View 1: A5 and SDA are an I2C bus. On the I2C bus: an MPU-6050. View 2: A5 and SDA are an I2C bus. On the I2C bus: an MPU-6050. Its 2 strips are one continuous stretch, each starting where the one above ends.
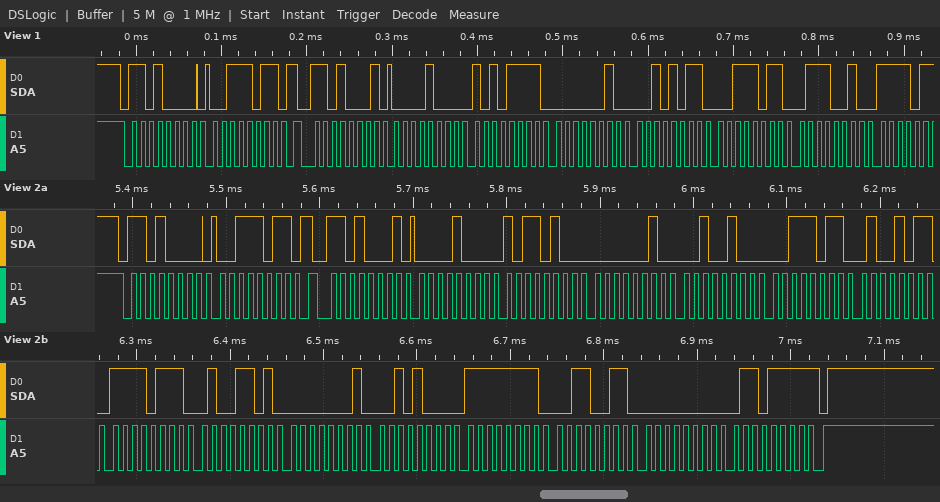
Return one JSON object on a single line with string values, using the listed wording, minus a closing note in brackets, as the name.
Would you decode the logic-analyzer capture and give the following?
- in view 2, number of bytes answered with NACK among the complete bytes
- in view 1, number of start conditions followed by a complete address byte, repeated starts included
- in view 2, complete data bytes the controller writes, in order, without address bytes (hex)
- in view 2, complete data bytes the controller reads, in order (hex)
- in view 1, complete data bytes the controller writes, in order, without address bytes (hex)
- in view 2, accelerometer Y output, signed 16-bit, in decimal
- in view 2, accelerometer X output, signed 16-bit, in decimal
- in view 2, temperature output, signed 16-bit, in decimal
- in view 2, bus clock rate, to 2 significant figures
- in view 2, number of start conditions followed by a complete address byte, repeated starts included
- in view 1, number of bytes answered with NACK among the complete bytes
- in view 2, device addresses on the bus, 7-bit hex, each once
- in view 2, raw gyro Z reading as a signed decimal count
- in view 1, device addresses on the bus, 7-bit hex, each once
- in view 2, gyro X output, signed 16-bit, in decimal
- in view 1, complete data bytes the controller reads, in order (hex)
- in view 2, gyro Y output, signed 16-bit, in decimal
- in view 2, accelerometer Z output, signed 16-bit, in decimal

{"in view 2, number of bytes answered with NACK among the complete bytes": "1", "in view 1, number of start conditions followed by a complete address byte, repeated starts included": "2", "in view 2, complete data bytes the controller writes, in order, without address bytes": "3B", "in view 2, complete data bytes the controller reads, in order": "08 B4 02 24 3B 4B F7 4D 01 28 FF 33 00 6F", "in view 1, complete data bytes the controller writes, in order, without address bytes": "3B", "in view 2, accelerometer Y output, signed 16-bit, in decimal": "548", "in view 2, accelerometer X output, signed 16-bit, in decimal": "2228", "in view 2, temperature output, signed 16-bit, in decimal": "-2227", "in view 2, bus clock rate, to 2 significant figures": "100 kHz", "in view 2, number of start conditions followed by a complete address byte, repeated starts included": "2", "in view 1, number of bytes answered with NACK among the complete bytes": "0", "in view 2, device addresses on the bus, 7-bit hex, each once": "0x68", "in view 2, raw gyro Z reading as a signed decimal count": "111", "in view 1, device addresses on the bus, 7-bit hex, each once": "0x68", "in view 2, gyro X output, signed 16-bit, in decimal": "296", "in view 1, complete data bytes the controller reads, in order": "08 AF 02 2B 3B 72", "in view 2, gyro Y output, signed 16-bit, in decimal": "-205", "in view 2, accelerometer Z output, signed 16-bit, in decimal": "15179"}
